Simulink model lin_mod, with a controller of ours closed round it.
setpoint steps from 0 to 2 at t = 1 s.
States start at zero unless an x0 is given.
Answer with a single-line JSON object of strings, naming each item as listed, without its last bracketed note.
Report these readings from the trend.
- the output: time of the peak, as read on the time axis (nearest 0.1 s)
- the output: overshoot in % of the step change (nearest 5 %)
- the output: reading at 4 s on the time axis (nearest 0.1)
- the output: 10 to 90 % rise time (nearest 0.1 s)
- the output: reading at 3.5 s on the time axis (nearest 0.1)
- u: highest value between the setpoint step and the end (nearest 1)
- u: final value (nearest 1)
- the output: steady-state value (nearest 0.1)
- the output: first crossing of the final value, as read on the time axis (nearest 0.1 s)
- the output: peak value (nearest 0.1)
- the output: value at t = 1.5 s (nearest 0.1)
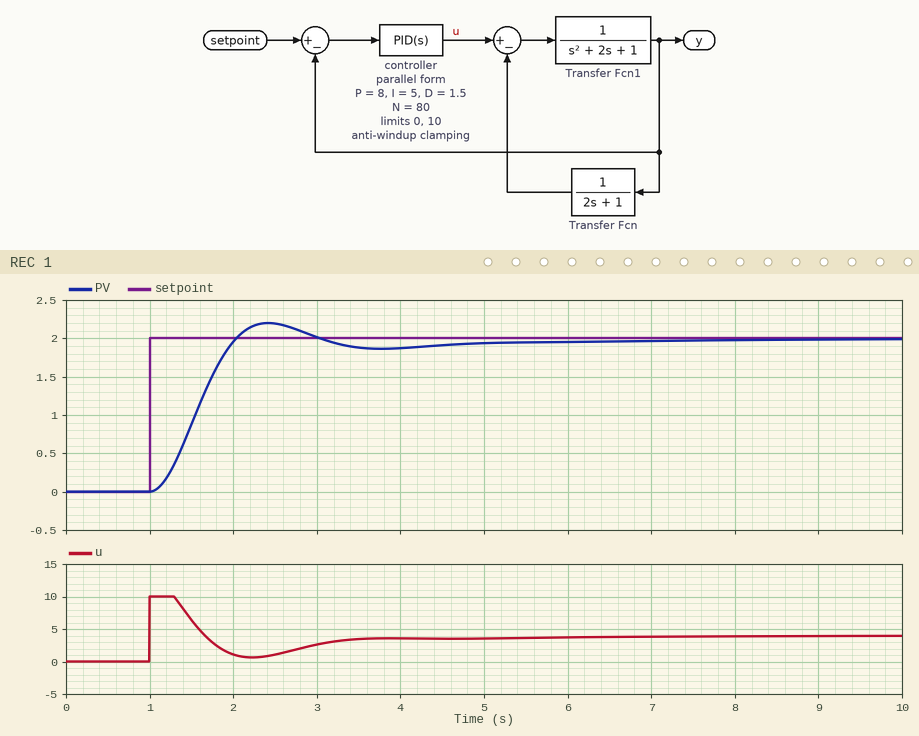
{"the output: time of the peak, as read on the time axis": "2.4 s", "the output: overshoot in % of the step change": "10 %", "the output: reading at 4 s on the time axis": "1.9", "the output: 10 to 90 % rise time": "0.7 s", "the output: reading at 3.5 s on the time axis": "1.9", "u: highest value between the setpoint step and the end": "10", "u: final value": "4", "the output: steady-state value": "2.0", "the output: first crossing of the final value, as read on the time axis": "2.0 s", "the output: peak value": "2.2", "the output: value at t = 1.5 s": "0.9"}
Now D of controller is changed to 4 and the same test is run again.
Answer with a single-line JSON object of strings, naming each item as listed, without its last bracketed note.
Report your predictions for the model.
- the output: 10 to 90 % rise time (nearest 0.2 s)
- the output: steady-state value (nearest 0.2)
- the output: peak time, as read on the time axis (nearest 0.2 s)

{"the output: 10 to 90 % rise time": "1.0 s", "the output: steady-state value": "2.0", "the output: peak time, as read on the time axis": "3.2 s"}
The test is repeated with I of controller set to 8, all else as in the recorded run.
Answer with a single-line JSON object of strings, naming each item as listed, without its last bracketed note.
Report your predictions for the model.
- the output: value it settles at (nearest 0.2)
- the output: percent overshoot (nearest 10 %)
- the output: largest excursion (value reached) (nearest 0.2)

{"the output: value it settles at": "2.0", "the output: percent overshoot": "20 %", "the output: largest excursion (value reached)": "2.4"}
